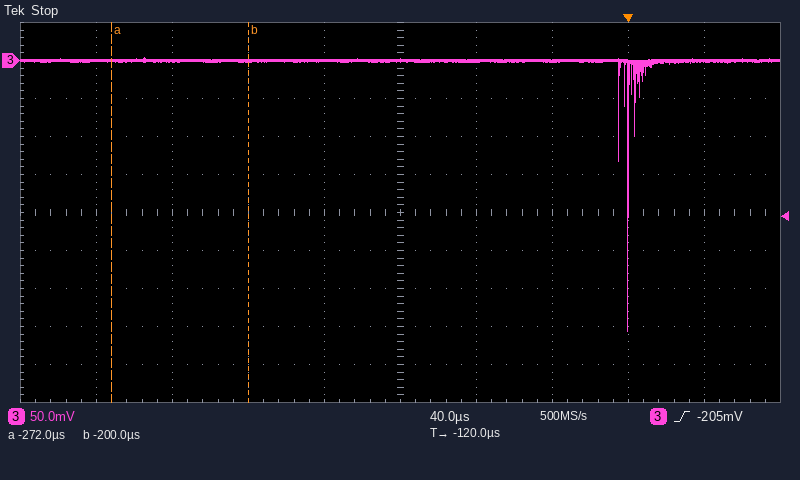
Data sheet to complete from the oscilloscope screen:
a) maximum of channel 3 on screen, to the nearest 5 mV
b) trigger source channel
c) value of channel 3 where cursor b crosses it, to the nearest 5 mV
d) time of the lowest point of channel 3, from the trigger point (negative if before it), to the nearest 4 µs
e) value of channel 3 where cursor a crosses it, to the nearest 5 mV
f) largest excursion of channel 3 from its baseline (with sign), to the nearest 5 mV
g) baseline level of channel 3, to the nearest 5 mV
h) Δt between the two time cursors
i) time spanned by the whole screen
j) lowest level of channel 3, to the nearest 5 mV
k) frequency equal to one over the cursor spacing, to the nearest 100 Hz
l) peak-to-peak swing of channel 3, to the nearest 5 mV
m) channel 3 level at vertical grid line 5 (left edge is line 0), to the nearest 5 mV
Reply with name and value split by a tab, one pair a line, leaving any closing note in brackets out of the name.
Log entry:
maximum of channel 3 on screen, to the nearest 5 mV	5 mV
trigger source channel	channel 3
value of channel 3 where cursor b crosses it, to the nearest 5 mV	0 mV
time of the lowest point of channel 3, from the trigger point (negative if before it), to the nearest 4 µs	0 µs
value of channel 3 where cursor a crosses it, to the nearest 5 mV	0 mV
largest excursion of channel 3 from its baseline (with sign), to the nearest 5 mV	-355 mV
baseline level of channel 3, to the nearest 5 mV	0 mV
Δt between the two time cursors	72 µs
time spanned by the whole screen	400 µs
lowest level of channel 3, to the nearest 5 mV	-355 mV
frequency equal to one over the cursor spacing, to the nearest 100 Hz	13.9 kHz
peak-to-peak swing of channel 3, to the nearest 5 mV	360 mV
channel 3 level at vertical grid line 5 (left edge is line 0), to the nearest 5 mV	0 mV
